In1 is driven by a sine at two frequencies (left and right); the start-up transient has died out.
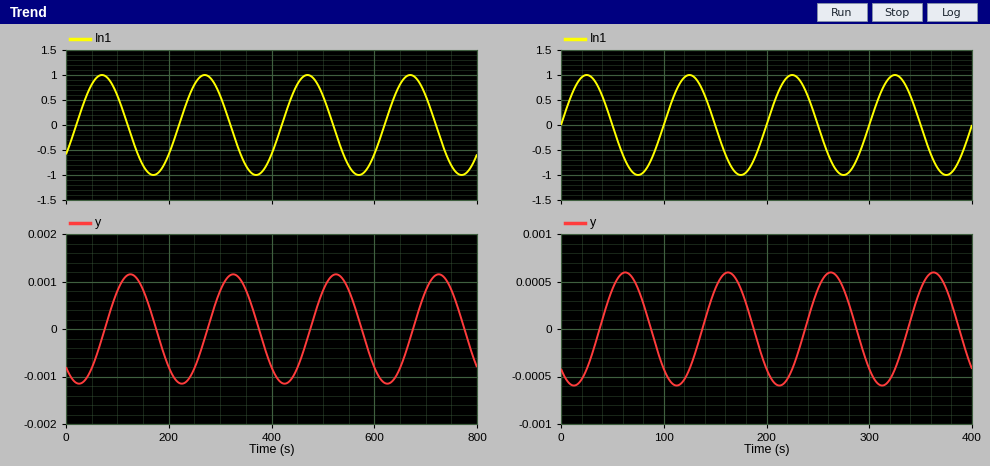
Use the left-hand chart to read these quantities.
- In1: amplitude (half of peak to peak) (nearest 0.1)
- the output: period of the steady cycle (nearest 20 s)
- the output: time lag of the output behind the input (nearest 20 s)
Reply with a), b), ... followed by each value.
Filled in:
a) 1.0
b) 200 s
c) 60 s
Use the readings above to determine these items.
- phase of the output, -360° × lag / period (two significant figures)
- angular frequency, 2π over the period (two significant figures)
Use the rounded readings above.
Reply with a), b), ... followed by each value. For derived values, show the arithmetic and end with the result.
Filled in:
a) -360 × 60 / 200 = -110°
b) 2π / 200 = 0.031 rad/s
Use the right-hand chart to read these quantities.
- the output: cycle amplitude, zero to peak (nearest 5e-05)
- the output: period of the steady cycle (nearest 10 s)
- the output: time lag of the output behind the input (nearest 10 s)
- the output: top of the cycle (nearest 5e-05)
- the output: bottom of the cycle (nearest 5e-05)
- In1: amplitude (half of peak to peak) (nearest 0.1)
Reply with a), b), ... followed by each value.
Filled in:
a) 0.00060
b) 100 s
c) 40 s
d) 0.00060
e) -0.00060
f) 1.0
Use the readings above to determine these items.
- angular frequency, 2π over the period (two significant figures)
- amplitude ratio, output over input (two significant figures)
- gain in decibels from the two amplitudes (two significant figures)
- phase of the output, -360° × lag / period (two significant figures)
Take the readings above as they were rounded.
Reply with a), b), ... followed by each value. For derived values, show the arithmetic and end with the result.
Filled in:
a) 2π / 100 = 0.063 rad/s
b) 0.0006 / 1 = 0.00060
c) 20 log10(0.0006 / 1) = -64 dB
d) -360 × 40 / 100 = -140°
